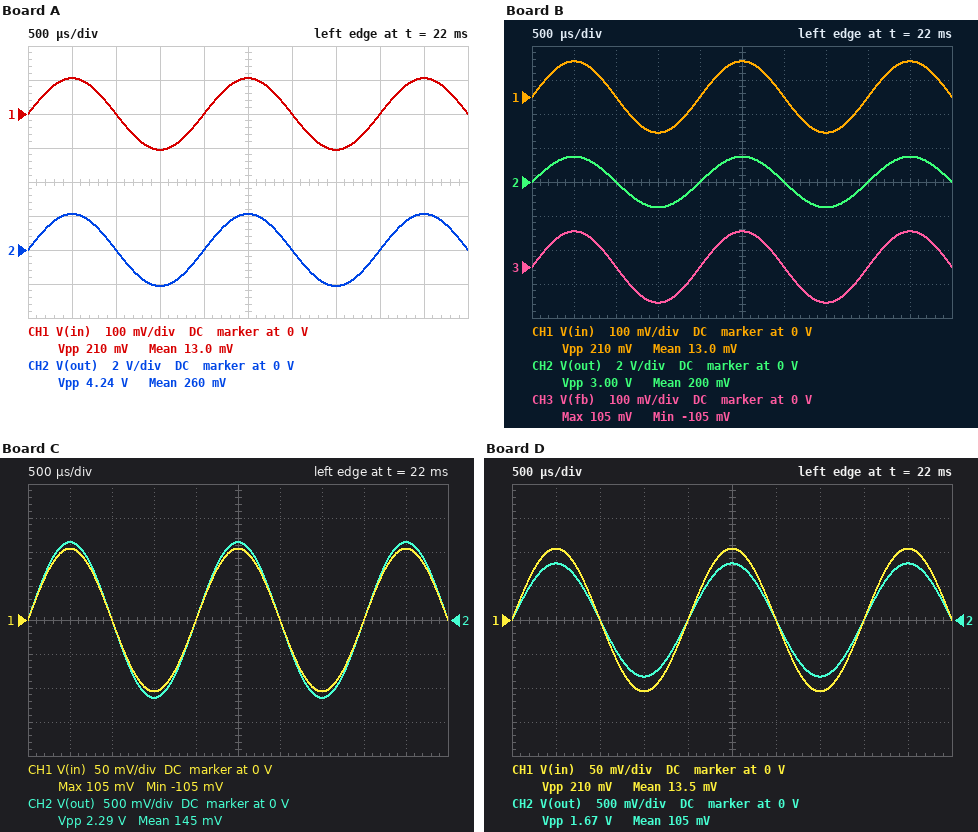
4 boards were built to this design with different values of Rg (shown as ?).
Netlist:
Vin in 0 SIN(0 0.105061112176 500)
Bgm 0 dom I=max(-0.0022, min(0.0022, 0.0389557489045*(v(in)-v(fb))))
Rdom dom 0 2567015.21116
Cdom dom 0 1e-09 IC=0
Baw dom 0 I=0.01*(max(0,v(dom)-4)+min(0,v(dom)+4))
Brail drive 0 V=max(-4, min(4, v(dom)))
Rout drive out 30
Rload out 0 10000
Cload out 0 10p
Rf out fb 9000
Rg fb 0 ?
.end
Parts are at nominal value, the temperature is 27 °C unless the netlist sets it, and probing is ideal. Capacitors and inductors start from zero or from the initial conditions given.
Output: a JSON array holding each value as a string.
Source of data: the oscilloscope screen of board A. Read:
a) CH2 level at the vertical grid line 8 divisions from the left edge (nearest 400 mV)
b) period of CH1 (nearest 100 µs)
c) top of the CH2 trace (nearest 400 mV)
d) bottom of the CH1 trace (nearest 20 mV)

["0 V", "2.0 ms", "2.0 V", "-100 mV"]
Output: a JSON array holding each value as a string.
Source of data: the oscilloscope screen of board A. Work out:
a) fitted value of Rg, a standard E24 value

["470 Ω"]
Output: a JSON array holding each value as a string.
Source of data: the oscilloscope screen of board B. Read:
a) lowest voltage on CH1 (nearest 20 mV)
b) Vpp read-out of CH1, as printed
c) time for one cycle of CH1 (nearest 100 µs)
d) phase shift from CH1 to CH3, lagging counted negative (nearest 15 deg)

["-100 mV", "210 mV", "2.0 ms", "0 deg"]
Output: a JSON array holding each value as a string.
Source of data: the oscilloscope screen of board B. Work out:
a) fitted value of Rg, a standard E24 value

["680 Ω"]
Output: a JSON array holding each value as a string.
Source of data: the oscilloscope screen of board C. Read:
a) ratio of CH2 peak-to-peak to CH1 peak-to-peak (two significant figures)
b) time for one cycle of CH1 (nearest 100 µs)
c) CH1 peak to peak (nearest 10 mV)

["11", "2.0 ms", "210 mV"]
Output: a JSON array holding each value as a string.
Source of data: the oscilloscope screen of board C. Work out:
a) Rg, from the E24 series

["910 Ω"]
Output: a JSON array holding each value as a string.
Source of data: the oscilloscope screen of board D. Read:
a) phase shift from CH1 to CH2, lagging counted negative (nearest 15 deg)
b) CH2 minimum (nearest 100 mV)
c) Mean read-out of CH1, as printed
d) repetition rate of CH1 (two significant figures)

["0 deg", "-800 mV", "13.5 mV", "500 Hz"]
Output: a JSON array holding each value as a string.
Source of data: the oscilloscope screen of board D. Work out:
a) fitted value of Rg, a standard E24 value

["1.3 kΩ"]
